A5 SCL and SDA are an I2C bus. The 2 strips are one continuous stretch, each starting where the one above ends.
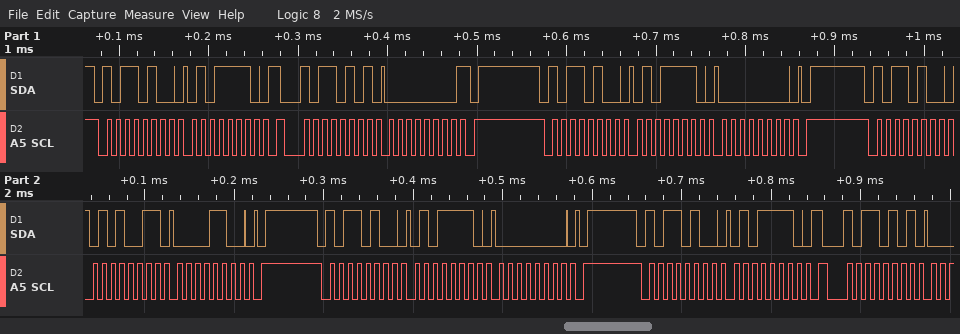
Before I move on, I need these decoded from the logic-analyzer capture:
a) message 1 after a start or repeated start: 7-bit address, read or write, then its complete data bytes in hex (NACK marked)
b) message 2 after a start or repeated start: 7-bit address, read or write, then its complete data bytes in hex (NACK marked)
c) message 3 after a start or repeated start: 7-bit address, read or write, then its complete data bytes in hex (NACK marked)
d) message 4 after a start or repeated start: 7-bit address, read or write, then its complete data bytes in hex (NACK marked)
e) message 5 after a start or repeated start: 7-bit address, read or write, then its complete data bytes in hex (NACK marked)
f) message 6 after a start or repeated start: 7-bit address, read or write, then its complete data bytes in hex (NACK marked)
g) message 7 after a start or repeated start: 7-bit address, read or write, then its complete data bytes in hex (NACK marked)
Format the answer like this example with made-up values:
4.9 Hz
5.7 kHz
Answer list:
0x5A write: 5E
0x5A read: 00 NACK
0x5A write: 5E 00
0x5A write: 53 0C
0x5A write: 5E 00
0x5A write: 5E
0x5A read
